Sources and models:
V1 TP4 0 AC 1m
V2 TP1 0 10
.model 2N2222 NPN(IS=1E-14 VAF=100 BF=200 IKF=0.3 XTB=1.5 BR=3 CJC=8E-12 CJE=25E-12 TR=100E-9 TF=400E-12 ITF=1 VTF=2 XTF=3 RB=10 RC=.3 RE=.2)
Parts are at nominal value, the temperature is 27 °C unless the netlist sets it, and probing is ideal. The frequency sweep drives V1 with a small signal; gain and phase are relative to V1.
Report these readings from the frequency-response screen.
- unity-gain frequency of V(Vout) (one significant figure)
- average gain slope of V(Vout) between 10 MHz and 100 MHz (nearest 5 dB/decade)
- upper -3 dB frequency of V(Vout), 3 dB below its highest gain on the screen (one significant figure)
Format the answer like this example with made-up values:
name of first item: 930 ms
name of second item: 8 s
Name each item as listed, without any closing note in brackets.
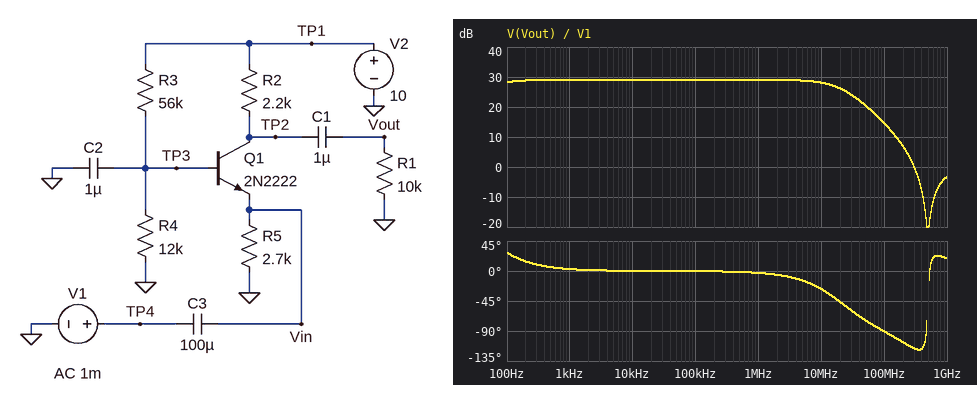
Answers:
unity-gain frequency of V(Vout): 300 MHz
average gain slope of V(Vout) between 10 MHz and 100 MHz: -15 dB/decade
upper -3 dB frequency of V(Vout), 3 dB below its highest gain on the screen: 20 MHz
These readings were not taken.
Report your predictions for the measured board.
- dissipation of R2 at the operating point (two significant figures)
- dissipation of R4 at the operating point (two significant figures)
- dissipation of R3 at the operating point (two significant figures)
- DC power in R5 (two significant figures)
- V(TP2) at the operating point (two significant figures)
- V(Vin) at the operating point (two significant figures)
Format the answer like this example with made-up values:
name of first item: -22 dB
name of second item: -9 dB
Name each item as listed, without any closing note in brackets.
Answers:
dissipation of R2 at the operating point: 370 µW
dissipation of R4 at the operating point: 250 µW
dissipation of R3 at the operating point: 1.2 mW
DC power in R5: 460 µW
V(TP2) at the operating point: 9.1 V
V(Vin) at the operating point: 1.1 V
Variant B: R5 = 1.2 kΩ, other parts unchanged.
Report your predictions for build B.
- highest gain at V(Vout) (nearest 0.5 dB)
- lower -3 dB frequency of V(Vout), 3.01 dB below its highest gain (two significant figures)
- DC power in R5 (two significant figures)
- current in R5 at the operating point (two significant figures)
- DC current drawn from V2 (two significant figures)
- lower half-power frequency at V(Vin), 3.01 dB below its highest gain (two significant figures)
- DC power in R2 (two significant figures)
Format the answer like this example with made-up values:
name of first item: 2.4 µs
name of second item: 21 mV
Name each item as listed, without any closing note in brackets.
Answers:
highest gain at V(Vout): 35.5 dB
lower -3 dB frequency of V(Vout), 3.01 dB below its highest gain: 86 Hz
DC power in R5: 960 µW
current in R5 at the operating point: 890 µA
DC current drawn from V2: 1.0 mA
lower half-power frequency at V(Vin), 3.01 dB below its highest gain: 65 Hz
DC power in R2: 1.7 mW
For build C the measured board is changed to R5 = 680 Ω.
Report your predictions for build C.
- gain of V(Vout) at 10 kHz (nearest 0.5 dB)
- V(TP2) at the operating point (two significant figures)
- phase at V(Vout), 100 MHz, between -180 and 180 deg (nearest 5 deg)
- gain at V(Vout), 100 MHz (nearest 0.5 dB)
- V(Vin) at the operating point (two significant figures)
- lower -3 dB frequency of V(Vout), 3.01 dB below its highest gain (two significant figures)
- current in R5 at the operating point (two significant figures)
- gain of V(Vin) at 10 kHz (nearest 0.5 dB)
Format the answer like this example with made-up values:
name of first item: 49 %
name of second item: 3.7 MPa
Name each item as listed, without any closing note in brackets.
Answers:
gain of V(Vout) at 10 kHz: 40.0 dB
V(TP2) at the operating point: 6.7 V
phase at V(Vout), 100 MHz, between -180 and 180 deg: -95 deg
gain at V(Vout), 100 MHz: 22.5 dB
V(Vin) at the operating point: 1.0 V
lower -3 dB frequency of V(Vout), 3.01 dB below its highest gain: 140 Hz
current in R5 at the operating point: 1.5 mA
gain of V(Vin) at 10 kHz: 0 dB
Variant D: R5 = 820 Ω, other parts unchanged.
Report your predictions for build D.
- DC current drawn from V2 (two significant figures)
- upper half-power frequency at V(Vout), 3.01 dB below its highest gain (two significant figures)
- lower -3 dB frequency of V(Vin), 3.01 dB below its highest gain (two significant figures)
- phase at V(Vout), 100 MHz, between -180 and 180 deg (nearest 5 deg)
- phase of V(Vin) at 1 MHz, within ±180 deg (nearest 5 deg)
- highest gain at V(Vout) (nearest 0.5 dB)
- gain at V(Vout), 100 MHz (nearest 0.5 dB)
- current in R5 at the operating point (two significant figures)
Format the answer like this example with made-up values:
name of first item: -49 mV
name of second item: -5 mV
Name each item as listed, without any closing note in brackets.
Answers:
DC current drawn from V2: 1.4 mA
upper half-power frequency at V(Vout), 3.01 dB below its highest gain: 15 MHz
lower -3 dB frequency of V(Vin), 3.01 dB below its highest gain: 95 Hz
phase at V(Vout), 100 MHz, between -180 and 180 deg: -95 deg
phase of V(Vin) at 1 MHz, within ±180 deg: 0 deg
highest gain at V(Vout): 38.5 dB
gain at V(Vout), 100 MHz: 21.5 dB
current in R5 at the operating point: 1.3 mA
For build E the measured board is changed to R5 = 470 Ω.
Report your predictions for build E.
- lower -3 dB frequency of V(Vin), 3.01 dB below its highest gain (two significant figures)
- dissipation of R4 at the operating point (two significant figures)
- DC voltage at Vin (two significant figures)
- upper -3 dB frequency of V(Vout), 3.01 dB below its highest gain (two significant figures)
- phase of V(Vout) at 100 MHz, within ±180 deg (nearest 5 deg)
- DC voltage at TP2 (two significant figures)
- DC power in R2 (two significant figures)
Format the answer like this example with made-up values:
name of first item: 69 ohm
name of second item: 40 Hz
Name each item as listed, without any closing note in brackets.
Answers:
lower -3 dB frequency of V(Vin), 3.01 dB below its highest gain: 160 Hz
dissipation of R4 at the operating point: 230 µW
DC voltage at Vin: 990 mV
upper -3 dB frequency of V(Vout), 3.01 dB below its highest gain: 11 MHz
phase of V(Vout) at 100 MHz, within ±180 deg: -95 deg
DC voltage at TP2: 5.4 V
DC power in R2: 9.7 mW
